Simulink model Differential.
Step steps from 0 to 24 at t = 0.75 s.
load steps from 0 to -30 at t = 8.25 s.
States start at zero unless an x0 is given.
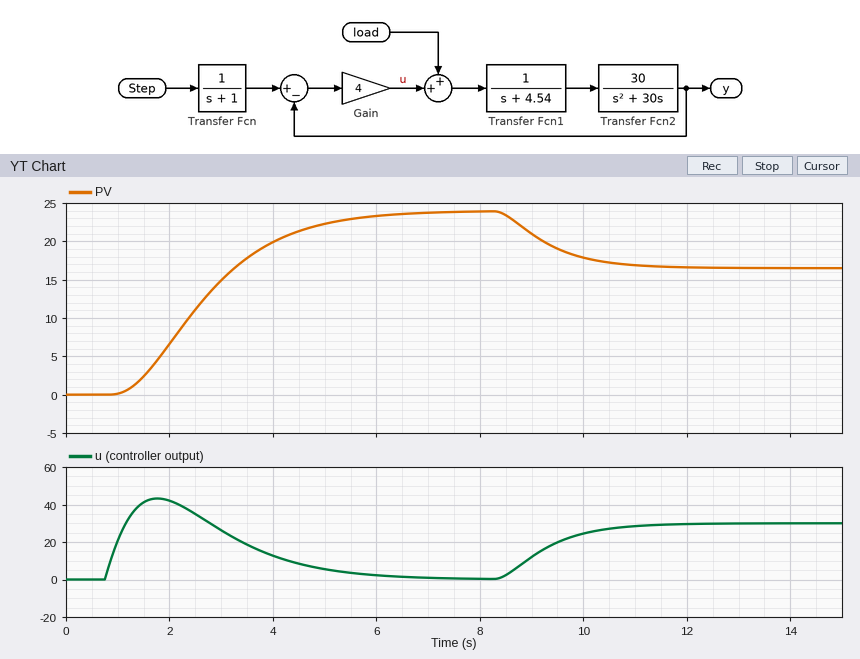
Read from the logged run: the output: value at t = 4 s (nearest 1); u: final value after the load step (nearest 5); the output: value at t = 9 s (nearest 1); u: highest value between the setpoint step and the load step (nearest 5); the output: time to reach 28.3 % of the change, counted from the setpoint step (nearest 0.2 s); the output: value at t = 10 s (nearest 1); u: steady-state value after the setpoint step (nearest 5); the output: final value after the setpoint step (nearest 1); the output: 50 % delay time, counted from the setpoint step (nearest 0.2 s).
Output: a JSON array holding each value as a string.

["20", "30", "21", "45", "1.2 s", "18", "0", "24", "1.8 s"]
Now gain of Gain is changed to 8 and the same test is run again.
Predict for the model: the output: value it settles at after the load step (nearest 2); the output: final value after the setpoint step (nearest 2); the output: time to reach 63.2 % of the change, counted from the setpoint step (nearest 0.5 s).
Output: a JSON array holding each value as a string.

["20", "24", "1.5 s"]
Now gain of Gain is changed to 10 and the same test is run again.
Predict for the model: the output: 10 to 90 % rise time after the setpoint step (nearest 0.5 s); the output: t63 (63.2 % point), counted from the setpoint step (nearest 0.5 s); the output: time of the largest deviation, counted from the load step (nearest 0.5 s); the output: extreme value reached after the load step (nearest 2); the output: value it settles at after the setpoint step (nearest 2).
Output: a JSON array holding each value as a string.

["2.0 s", "1.5 s", "1.5 s", "20", "24"]
